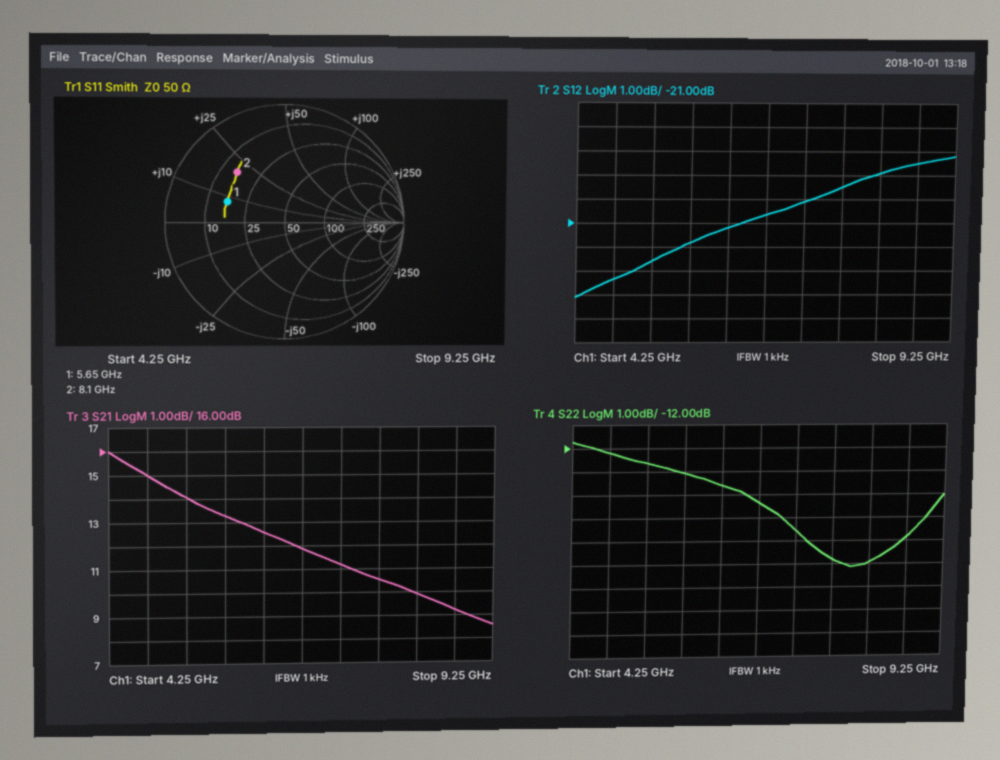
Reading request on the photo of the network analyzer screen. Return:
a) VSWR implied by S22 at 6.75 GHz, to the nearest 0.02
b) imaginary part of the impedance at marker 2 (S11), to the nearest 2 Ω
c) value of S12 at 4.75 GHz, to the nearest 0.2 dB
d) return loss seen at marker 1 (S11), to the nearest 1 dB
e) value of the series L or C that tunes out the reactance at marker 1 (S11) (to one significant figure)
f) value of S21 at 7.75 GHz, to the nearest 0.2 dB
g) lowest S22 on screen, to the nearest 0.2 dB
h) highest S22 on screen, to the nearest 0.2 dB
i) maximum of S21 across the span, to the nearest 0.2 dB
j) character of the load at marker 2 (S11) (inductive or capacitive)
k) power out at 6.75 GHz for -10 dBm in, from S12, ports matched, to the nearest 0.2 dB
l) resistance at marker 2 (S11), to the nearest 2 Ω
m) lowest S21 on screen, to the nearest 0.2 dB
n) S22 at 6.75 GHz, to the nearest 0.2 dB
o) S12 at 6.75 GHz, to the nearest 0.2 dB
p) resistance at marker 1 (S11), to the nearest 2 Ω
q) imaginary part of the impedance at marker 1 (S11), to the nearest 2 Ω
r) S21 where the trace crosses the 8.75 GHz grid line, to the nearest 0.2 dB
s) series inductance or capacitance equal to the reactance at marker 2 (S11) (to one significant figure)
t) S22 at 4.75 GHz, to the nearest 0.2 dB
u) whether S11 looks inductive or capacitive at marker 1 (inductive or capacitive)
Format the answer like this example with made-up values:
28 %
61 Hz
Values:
1.48
+20 Ω
-23.4 dB
6 dB
4 pF
10.6 dB
-17.2 dB
-11.8 dB
16.0 dB
inductive
-30.6 dBm
16 Ω
8.6 dB
-14.4 dB
-20.6 dB
16 Ω
+8 Ω
9.2 dB
400 pH
-12.2 dB
inductive
